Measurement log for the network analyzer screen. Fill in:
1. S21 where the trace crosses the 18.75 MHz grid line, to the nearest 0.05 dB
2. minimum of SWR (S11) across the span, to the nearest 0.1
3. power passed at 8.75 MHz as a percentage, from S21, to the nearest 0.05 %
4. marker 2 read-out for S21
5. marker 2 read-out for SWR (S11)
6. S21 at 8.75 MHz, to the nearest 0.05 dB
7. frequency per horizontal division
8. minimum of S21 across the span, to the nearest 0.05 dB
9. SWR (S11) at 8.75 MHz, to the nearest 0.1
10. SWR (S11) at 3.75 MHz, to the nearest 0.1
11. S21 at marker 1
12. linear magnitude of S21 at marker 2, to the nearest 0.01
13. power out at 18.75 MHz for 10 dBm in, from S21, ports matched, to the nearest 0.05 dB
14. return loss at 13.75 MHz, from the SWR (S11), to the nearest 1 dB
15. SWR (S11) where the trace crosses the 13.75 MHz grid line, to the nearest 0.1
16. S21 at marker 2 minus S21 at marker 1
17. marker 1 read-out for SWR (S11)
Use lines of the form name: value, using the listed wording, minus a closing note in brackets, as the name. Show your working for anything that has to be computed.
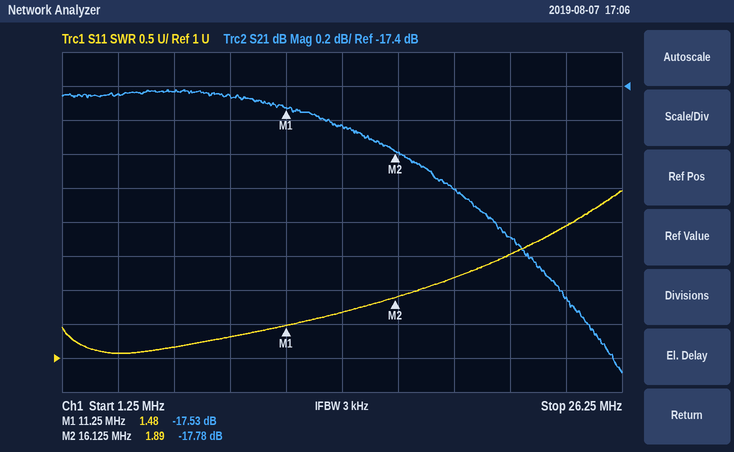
S21 where the trace crosses the 18.75 MHz grid line, to the nearest 0.05 dB: -18.00 dB
minimum of SWR (S11) across the span, to the nearest 0.1: 1.1
power passed at 8.75 MHz as a percentage, from S21, to the nearest 0.05 %: 10^(-17.45/10) ≈ 1.80 %
marker 2 read-out for S21: -17.78 dB
marker 2 read-out for SWR: 1.89
S21 at 8.75 MHz, to the nearest 0.05 dB: -17.45 dB
frequency per horizontal division: 2.5 MHz
minimum of S21 across the span, to the nearest 0.05 dB: -19.10 dB
SWR (S11) at 8.75 MHz, to the nearest 0.1: 1.3
SWR (S11) at 3.75 MHz, to the nearest 0.1: 1.1
S21 at marker 1: -17.53 dB
linear magnitude of S21 at marker 2, to the nearest 0.01: 10^(-17.78/20) ≈ 0.13
power out at 18.75 MHz for 10 dBm in, from S21, ports matched, to the nearest 0.05 dB: 10 dBm + (-18.00 dB) = -8.00 dBm
return loss at 13.75 MHz, from the SWR (S11), to the nearest 1 dB: −20 log10((1.7 − 1)/(1.7 + 1)) ≈ 12 dB
SWR (S11) where the trace crosses the 13.75 MHz grid line, to the nearest 0.1: 1.7
S21 at marker 2 minus S21 at marker 1: -17.78 − (-17.53) = -0.25 dB
marker 1 read-out for SWR: 1.48
